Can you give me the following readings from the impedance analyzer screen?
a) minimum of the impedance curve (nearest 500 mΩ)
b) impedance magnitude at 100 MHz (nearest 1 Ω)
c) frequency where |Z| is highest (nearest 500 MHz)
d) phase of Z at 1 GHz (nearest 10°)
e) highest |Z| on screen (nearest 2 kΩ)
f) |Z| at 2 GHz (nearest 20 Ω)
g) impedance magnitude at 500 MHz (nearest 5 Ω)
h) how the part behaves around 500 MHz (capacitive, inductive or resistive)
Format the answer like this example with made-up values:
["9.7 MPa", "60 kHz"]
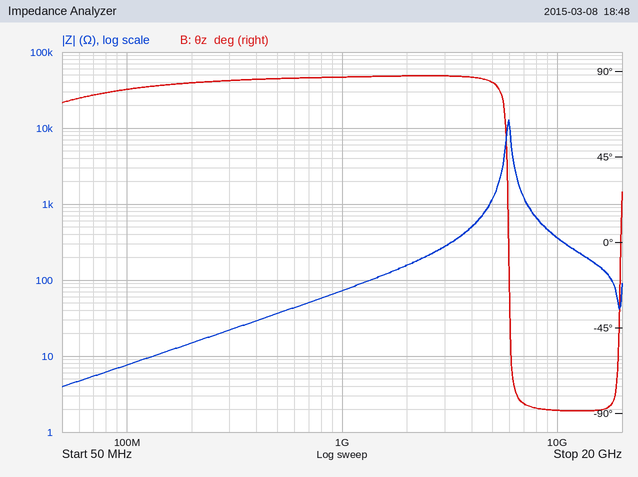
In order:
["4.0 Ω", "8 Ω", "6.0 GHz", "90°", "12 kΩ", "160 Ω", "35 Ω", "inductive"]
